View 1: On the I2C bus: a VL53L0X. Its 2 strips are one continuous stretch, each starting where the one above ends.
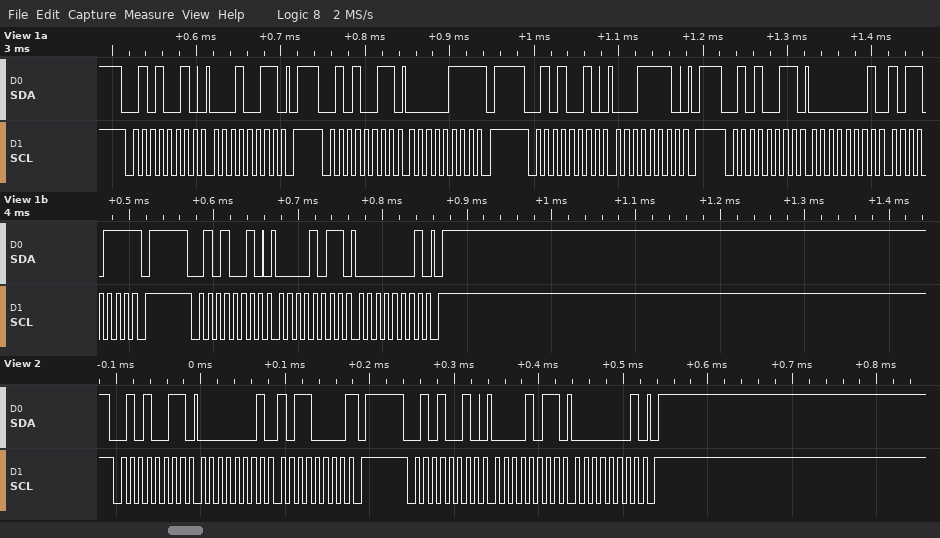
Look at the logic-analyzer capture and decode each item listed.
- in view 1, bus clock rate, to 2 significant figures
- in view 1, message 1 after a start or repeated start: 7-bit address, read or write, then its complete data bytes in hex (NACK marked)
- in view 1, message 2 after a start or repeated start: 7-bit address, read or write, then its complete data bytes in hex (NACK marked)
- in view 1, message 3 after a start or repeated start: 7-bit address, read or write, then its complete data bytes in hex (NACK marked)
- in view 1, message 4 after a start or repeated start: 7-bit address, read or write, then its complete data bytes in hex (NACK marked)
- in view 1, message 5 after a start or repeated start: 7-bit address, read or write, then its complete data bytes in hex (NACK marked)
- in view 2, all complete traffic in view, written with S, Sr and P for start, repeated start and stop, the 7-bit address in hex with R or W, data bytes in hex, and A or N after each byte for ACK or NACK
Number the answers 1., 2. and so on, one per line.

1. 100 kHz
2. 0x29 write: 13
3. 0x29 read: 07 NACK
4. 0x29 write: 1E
5. 0x29 read: 01 B7 NACK
6. 0x29 write: 0B 01
7. S 29R A 01 A B0 N P S 29W A 0B A 01 A P
